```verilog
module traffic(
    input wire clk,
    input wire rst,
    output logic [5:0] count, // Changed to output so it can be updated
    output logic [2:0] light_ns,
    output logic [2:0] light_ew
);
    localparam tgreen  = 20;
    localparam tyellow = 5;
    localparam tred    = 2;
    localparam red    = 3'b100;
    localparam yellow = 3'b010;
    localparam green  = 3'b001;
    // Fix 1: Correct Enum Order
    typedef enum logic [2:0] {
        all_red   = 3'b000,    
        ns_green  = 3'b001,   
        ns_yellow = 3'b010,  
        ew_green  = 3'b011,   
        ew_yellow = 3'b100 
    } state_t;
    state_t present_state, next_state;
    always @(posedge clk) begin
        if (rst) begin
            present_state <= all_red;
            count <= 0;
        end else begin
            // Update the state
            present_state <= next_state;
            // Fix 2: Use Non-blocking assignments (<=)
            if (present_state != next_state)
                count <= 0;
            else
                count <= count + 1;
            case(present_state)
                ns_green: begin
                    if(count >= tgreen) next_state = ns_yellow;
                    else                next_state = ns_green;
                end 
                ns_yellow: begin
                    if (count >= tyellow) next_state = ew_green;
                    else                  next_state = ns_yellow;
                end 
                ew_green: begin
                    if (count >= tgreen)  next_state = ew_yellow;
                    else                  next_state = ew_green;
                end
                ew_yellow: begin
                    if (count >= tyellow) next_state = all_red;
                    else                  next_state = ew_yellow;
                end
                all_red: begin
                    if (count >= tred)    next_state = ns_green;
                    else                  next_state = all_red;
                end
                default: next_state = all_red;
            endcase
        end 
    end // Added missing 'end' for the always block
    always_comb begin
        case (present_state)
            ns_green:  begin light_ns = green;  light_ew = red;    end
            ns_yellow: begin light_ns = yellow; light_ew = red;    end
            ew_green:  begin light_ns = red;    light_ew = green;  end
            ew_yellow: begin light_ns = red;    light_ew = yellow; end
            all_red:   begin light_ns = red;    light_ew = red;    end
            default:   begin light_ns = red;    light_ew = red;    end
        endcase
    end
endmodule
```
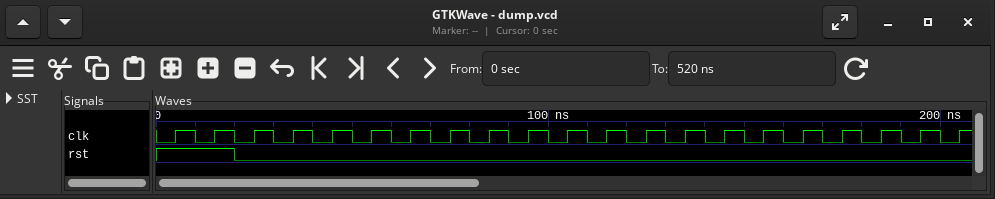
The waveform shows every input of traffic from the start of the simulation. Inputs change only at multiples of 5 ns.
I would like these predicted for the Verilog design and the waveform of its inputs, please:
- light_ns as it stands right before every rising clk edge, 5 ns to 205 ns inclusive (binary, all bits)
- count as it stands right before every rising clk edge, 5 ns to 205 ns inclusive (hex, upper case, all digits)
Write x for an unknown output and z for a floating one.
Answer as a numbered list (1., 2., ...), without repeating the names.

1. 100, 100, 100, 100, 100, 100, 001, 001, 001, 001, 001, 001, 001, 001, 001, 001, 001, 001, 001, 001, 001
2. x, 00, 00, 01, 02, 03, 00, 01, 02, 03, 04, 05, 06, 07, 08, 09, 0A, 0B, 0C, 0D, 0E
